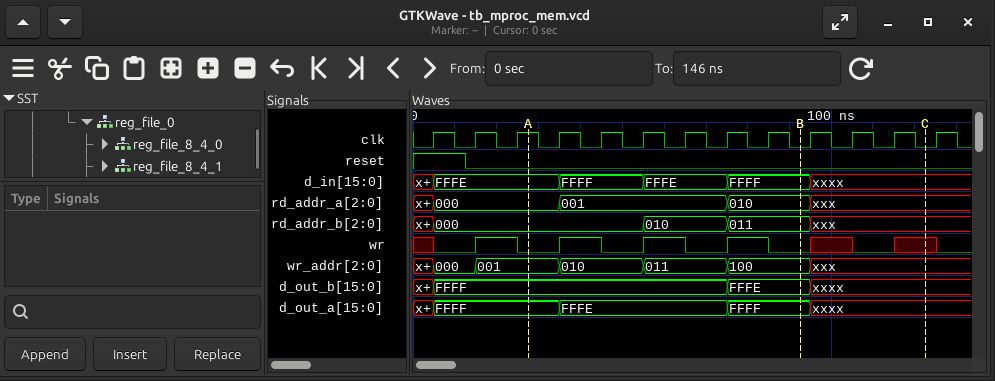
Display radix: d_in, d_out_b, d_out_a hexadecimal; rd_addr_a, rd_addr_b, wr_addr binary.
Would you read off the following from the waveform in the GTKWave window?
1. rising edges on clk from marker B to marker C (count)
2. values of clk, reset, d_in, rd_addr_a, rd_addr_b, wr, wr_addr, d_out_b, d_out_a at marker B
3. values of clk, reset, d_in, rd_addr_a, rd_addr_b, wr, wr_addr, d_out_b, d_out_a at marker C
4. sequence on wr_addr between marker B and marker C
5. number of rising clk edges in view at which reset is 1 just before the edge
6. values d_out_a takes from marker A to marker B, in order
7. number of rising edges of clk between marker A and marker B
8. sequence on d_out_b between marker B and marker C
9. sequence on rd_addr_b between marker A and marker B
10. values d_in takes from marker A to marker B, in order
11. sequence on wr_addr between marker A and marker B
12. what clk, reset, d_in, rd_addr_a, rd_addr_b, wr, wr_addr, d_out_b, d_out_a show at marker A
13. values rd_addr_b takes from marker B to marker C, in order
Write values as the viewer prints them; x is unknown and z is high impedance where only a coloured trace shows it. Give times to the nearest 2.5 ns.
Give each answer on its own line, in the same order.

3
clk=0, reset=0, d_in=FFFF, rd_addr_a=010, rd_addr_b=011, wr=0, wr_addr=100, d_out_b=FFFE, d_out_a=FFFF
clk=0, reset=0, d_in=xxxx, rd_addr_a=xxx, rd_addr_b=xxx, wr=x, wr_addr=xxx, d_out_b=xxxx, d_out_a=xxxx
100, xxx
1
FFFF, FFFE, FFFF
6
FFFE, xxxx
000, 010, 011
FFFE, FFFF, FFFE, FFFF
001, 010, 011, 100
clk=1, reset=0, d_in=FFFE, rd_addr_a=000, rd_addr_b=000, wr=0, wr_addr=001, d_out_b=FFFF, d_out_a=FFFF
011, xxx
